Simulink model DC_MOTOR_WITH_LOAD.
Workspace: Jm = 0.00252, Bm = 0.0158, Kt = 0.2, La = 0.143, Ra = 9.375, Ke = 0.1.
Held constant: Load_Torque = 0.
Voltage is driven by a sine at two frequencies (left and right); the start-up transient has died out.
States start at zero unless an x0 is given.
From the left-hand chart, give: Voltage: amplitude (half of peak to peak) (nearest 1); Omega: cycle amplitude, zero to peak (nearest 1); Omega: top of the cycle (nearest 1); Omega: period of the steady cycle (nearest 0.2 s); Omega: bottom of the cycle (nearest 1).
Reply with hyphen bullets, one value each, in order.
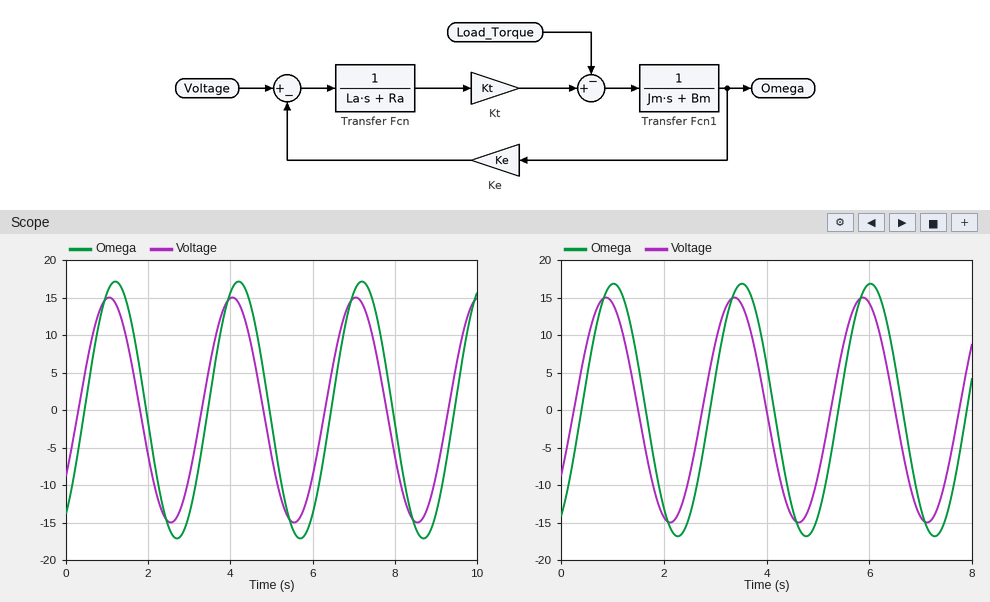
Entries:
- 15
- 17
- 17
- 3.0 s
- -17
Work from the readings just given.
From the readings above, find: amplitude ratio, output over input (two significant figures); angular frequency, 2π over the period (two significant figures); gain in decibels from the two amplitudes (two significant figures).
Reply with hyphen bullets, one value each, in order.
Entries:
- 1.1
- 2.1 rad/s
- 1.1 dB
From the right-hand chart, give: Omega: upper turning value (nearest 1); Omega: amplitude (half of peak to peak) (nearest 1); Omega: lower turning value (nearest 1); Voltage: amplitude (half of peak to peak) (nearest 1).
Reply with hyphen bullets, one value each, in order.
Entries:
- 17
- 17
- -17
- 15
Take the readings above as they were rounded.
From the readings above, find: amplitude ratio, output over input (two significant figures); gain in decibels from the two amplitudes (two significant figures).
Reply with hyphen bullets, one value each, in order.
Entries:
- 1.1
- 1.1 dB
